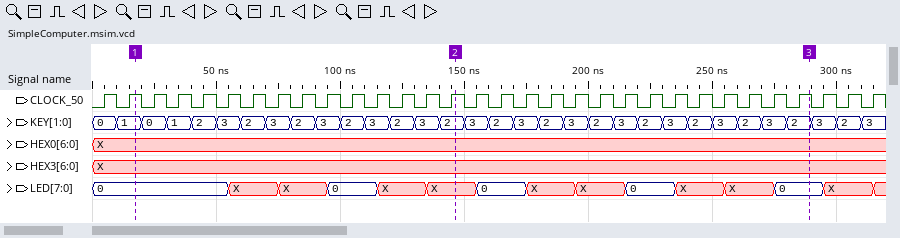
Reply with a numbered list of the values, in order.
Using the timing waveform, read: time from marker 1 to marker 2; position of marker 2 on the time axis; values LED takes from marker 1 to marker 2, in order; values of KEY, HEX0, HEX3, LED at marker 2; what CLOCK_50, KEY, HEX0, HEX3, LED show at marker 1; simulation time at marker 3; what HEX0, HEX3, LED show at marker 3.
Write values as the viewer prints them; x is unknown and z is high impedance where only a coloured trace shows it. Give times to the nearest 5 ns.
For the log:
1. 130 ns
2. 145 ns
3. 0, X, X, 0, X, X
4. KEY=2, HEX0=X, HEX3=X, LED=X
5. CLOCK_50=1, KEY=1, HEX0=X, HEX3=X, LED=0
6. 290 ns
7. HEX0=X, HEX3=X, LED=0
